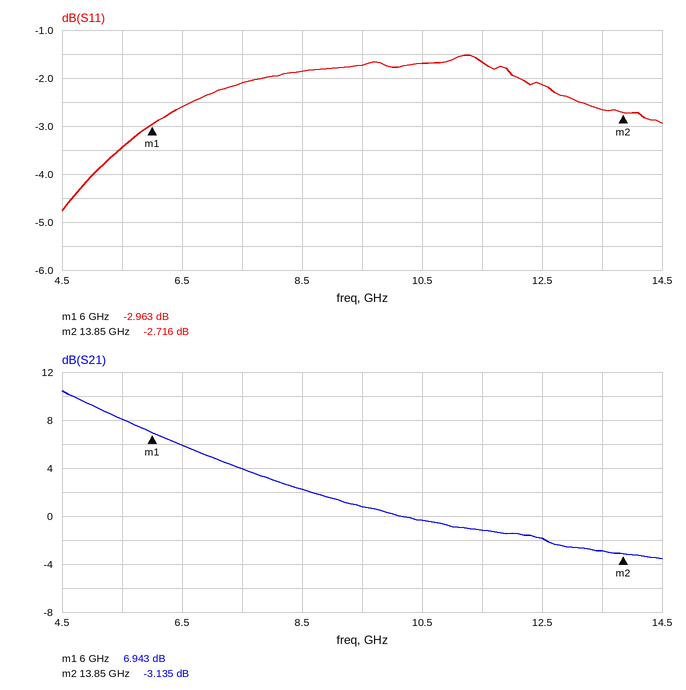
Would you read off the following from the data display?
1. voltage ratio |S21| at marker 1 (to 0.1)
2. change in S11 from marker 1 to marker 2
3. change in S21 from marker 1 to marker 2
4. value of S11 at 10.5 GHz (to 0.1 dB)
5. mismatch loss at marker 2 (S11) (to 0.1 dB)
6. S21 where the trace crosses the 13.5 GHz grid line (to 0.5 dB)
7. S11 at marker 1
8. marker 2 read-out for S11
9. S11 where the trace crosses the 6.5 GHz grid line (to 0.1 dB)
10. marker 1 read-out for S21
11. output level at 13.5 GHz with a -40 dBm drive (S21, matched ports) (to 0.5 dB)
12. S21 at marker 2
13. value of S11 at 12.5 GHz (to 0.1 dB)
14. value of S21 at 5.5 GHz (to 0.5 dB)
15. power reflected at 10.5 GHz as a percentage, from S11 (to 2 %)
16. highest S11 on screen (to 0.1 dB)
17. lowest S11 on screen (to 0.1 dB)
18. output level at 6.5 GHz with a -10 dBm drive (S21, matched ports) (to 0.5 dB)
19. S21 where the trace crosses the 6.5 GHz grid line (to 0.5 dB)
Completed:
2.2
0.247 dB
-10.078 dB
-1.7 dB
3.3 dB
-3.0 dB
-2.963 dB
-2.716 dB
-2.6 dB
6.943 dB
-43.0 dBm
-3.135 dB
-2.1 dB
8.0 dB
68 %
-1.5 dB
-4.8 dB
-4.0 dBm
6.0 dB
